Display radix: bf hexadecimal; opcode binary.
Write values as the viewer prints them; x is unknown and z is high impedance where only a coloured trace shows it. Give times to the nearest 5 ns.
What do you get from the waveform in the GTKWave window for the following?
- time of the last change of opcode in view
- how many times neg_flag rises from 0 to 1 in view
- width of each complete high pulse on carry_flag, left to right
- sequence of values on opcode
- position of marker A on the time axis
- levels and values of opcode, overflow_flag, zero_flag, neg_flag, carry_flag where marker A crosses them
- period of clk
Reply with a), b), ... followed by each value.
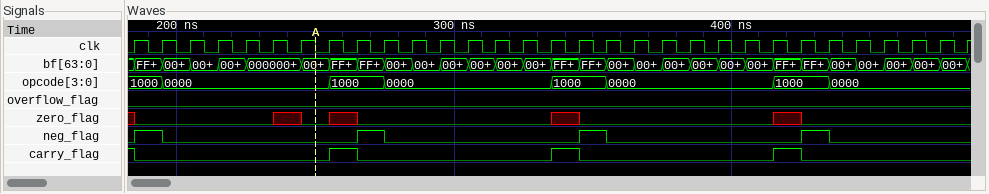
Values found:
a) 435 ns
b) 4
c) 10 ns, 10 ns, 10 ns
d) 1000, 0000, 1000, 0000, 1000, 0000, 1000, 0000
e) 250 ns
f) opcode=0000, overflow_flag=0, zero_flag=0, neg_flag=0, carry_flag=0
g) 10 ns
